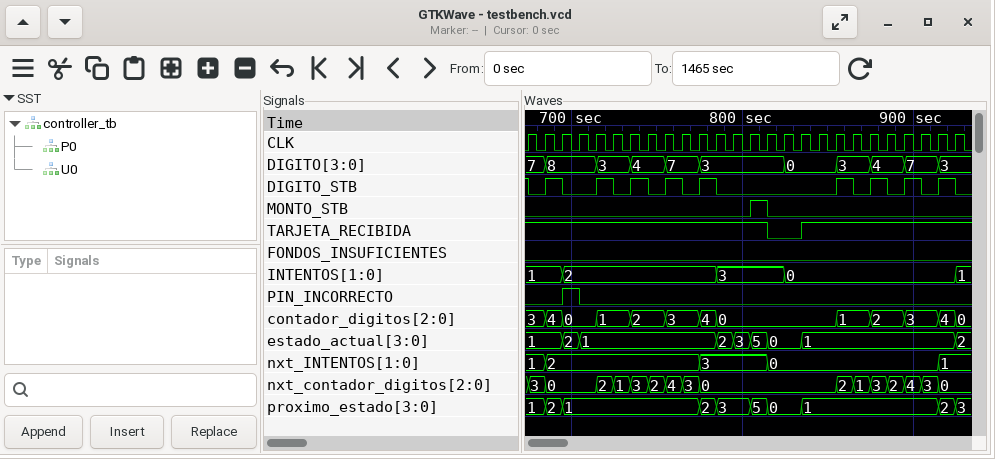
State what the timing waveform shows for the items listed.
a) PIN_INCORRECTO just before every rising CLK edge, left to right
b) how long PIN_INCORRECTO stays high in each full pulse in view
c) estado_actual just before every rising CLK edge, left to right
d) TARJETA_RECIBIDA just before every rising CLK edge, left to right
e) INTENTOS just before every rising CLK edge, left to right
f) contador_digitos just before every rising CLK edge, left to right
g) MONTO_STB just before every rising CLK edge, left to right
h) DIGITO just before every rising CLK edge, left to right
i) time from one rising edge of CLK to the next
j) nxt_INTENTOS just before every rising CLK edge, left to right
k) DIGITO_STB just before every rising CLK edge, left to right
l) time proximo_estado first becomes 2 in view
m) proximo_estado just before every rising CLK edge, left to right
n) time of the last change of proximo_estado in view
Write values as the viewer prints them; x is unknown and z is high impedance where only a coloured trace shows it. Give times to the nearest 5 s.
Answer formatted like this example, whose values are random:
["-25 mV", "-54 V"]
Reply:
["0 0 0 1 0 0 0 0 0 0 0 0 0 0 0 0 0 0 0 0 0 0 0 0 0 0", "10 s", "1, 1, 1, 2, 1, 1, 1, 1, 1, 1, 1, 1, 2, 3, 5, 0, 0, 1, 1, 1, 1, 1, 1, 1, 1, 1", "1 1 1 1 1 1 1 1 1 1 1 1 1 1 1 0 0 1 1 1 1 1 1 1 1 1", "1, 1, 1, 2, 2, 2, 2, 2, 2, 2, 2, 2, 3, 3, 3, 3, 0, 0, 0, 0, 0, 0, 0, 0, 0, 0", "3, 3, 4, 0, 0, 1, 1, 2, 2, 3, 3, 4, 0, 0, 0, 0, 0, 0, 0, 1, 1, 2, 2, 3, 3, 4", "0 0 0 0 0 0 0 0 0 0 0 0 0 0 1 0 0 0 0 0 0 0 0 0 0 0", "7, 7, 8, 8, 8, 3, 3, 4, 4, 7, 7, 3, 3, 3, 3, 3, 0, 0, 0, 3, 3, 4, 4, 7, 7, 3", "10 s", "1, 1, 2, 2, 2, 2, 2, 2, 2, 2, 2, 3, 3, 3, 3, 0, 0, 0, 0, 0, 0, 0, 0, 0, 0, 1", "1 0 1 0 0 1 0 1 0 1 0 1 0 0 0 0 0 0 0 1 0 1 0 1 0 1", "685 s", "1, 1, 2, 1, 1, 1, 1, 1, 1, 1, 1, 2, 3, 3, 5, 0, 0, 1, 1, 1, 1, 1, 1, 1, 1, 2", "925 s"]
